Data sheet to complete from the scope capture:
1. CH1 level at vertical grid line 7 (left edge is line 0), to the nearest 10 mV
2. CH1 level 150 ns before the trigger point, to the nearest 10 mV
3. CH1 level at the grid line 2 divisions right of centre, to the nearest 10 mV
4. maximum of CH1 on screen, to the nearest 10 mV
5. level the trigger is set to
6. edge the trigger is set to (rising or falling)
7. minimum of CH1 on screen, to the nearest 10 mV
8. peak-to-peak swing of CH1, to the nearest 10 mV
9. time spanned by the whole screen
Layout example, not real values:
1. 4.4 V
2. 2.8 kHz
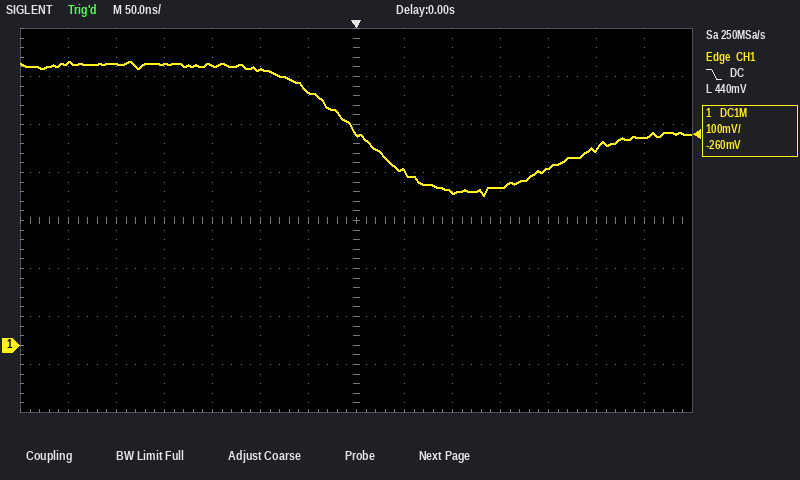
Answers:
1. 440 mV
2. 580 mV
3. 320 mV
4. 590 mV
5. 440 mV
6. falling
7. 310 mV
8. 280 mV
9. 700 ns
